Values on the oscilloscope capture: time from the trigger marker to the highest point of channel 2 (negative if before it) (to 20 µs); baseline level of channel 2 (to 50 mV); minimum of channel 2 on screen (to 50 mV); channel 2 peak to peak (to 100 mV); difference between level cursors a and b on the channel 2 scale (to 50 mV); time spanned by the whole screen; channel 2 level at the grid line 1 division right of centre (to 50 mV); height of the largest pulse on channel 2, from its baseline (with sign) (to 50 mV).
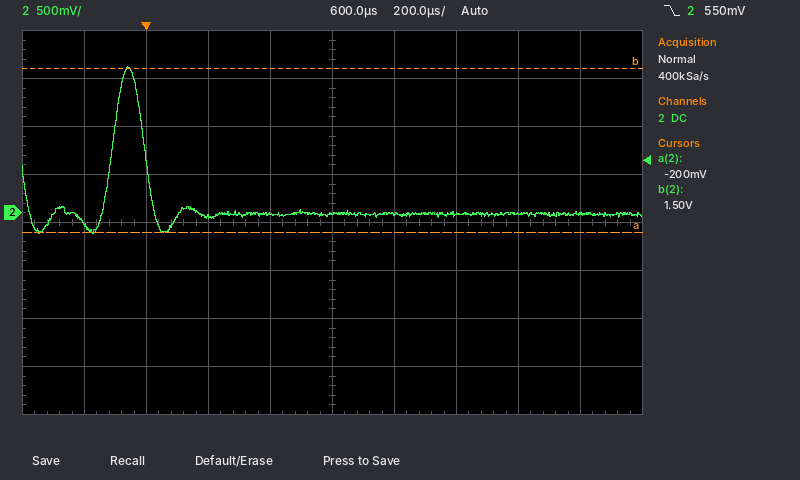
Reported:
-60 µs
0 mV
-200 mV
1.70 V
1.70 V
2 ms
0 mV
+1.55 V
